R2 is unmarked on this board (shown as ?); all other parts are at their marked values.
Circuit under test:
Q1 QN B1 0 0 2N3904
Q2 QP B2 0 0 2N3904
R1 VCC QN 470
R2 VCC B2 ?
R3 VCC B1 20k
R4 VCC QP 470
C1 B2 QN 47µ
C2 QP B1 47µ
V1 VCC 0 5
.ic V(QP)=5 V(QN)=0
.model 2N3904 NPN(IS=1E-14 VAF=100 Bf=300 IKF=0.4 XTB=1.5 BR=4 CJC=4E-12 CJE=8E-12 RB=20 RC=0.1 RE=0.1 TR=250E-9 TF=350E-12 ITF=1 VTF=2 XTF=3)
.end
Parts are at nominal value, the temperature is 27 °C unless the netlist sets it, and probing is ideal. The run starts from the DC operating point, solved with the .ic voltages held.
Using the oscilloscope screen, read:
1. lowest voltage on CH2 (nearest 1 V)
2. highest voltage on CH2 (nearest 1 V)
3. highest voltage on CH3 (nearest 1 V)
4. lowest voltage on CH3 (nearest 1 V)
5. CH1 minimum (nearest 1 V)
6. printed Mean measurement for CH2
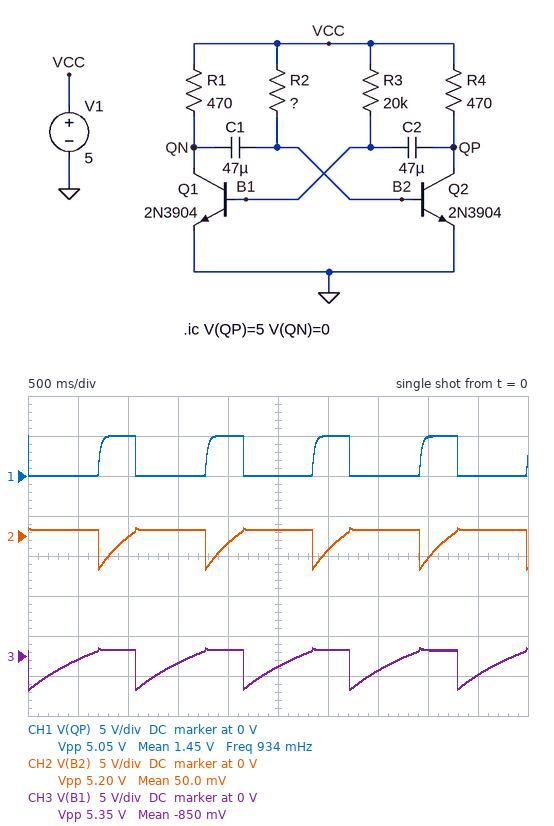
-4 V
1 V
1 V
-4 V
0 V
50.0 mV
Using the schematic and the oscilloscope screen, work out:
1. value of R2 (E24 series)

11 kΩ
